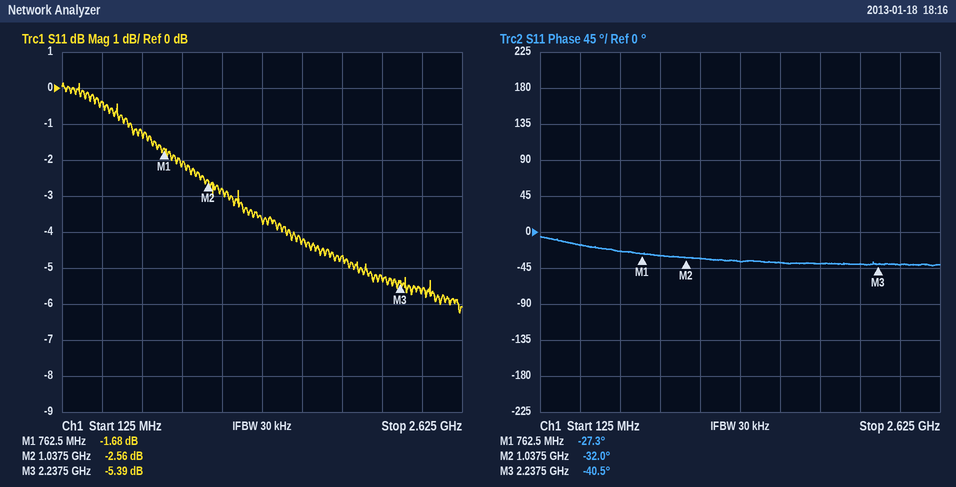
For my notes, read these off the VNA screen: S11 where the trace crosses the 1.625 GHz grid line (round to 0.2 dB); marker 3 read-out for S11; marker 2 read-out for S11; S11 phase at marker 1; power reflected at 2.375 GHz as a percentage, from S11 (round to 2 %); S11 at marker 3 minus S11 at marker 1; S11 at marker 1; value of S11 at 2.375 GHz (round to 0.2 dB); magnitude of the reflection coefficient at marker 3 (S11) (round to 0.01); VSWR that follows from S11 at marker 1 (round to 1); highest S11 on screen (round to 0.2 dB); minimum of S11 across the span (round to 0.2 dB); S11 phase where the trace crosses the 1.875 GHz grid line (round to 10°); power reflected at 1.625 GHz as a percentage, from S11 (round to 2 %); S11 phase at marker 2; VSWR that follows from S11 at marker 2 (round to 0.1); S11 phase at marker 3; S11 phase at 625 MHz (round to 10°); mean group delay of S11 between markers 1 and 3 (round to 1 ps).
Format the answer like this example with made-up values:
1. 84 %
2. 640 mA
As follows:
1. -4.2 dB
2. -5.39 dB
3. -2.56 dB
4. -27.3°
5. 28 %
6. -3.71 dB
7. -1.68 dB
8. -5.6 dB
9. 0.54
10. 10
11. 0.2 dB
12. -6.2 dB
13. -40°
14. 38 %
15. -32.0°
16. 6.8
17. -40.5°
18. -20°
19. 25 ps
